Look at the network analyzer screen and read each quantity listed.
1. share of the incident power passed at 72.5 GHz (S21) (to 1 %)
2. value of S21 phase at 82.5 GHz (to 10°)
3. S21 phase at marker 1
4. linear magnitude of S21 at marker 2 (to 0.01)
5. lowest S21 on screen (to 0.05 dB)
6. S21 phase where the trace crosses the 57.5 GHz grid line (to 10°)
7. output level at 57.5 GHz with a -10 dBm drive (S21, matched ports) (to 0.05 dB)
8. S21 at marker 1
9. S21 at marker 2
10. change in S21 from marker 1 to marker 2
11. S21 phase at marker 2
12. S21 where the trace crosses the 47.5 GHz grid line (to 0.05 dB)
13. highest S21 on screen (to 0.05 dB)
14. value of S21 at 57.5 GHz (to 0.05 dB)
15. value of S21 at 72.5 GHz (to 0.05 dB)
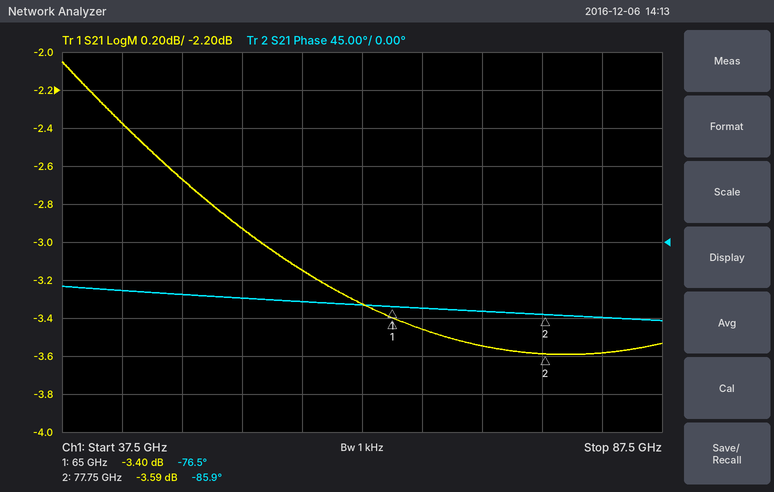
44 %
-90°
-76.5°
0.66
-3.60 dB
-70°
-13.15 dBm
-3.40 dB
-3.59 dB
-0.19 dB
-85.9°
-2.65 dB
-2.05 dB
-3.15 dB
-3.55 dB
